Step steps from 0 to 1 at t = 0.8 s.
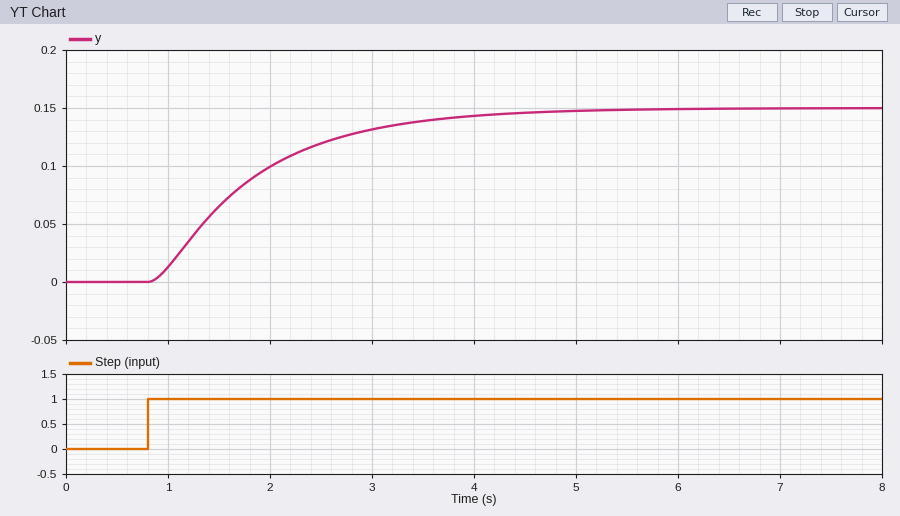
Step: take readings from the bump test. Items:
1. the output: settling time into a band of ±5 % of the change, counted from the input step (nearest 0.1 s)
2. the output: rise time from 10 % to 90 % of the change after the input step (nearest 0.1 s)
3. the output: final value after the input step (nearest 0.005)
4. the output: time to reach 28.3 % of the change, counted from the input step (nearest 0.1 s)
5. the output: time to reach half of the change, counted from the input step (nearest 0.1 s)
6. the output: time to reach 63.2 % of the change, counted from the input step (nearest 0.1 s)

3.1 s
2.2 s
0.150
0.5 s
0.8 s
1.1 s
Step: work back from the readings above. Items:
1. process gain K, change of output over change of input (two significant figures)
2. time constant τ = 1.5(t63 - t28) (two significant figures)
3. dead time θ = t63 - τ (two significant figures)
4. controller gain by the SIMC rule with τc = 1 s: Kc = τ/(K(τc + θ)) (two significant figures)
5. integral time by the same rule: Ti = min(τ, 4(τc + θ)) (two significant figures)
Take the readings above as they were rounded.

0.15
0.90 s
0.20 s
5.0
0.90 s
